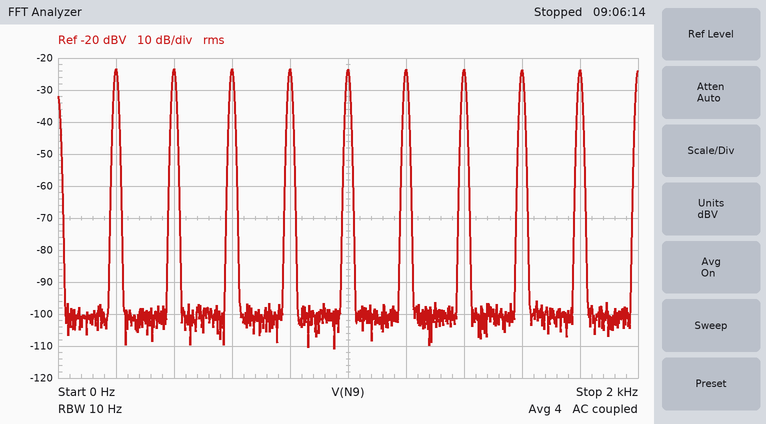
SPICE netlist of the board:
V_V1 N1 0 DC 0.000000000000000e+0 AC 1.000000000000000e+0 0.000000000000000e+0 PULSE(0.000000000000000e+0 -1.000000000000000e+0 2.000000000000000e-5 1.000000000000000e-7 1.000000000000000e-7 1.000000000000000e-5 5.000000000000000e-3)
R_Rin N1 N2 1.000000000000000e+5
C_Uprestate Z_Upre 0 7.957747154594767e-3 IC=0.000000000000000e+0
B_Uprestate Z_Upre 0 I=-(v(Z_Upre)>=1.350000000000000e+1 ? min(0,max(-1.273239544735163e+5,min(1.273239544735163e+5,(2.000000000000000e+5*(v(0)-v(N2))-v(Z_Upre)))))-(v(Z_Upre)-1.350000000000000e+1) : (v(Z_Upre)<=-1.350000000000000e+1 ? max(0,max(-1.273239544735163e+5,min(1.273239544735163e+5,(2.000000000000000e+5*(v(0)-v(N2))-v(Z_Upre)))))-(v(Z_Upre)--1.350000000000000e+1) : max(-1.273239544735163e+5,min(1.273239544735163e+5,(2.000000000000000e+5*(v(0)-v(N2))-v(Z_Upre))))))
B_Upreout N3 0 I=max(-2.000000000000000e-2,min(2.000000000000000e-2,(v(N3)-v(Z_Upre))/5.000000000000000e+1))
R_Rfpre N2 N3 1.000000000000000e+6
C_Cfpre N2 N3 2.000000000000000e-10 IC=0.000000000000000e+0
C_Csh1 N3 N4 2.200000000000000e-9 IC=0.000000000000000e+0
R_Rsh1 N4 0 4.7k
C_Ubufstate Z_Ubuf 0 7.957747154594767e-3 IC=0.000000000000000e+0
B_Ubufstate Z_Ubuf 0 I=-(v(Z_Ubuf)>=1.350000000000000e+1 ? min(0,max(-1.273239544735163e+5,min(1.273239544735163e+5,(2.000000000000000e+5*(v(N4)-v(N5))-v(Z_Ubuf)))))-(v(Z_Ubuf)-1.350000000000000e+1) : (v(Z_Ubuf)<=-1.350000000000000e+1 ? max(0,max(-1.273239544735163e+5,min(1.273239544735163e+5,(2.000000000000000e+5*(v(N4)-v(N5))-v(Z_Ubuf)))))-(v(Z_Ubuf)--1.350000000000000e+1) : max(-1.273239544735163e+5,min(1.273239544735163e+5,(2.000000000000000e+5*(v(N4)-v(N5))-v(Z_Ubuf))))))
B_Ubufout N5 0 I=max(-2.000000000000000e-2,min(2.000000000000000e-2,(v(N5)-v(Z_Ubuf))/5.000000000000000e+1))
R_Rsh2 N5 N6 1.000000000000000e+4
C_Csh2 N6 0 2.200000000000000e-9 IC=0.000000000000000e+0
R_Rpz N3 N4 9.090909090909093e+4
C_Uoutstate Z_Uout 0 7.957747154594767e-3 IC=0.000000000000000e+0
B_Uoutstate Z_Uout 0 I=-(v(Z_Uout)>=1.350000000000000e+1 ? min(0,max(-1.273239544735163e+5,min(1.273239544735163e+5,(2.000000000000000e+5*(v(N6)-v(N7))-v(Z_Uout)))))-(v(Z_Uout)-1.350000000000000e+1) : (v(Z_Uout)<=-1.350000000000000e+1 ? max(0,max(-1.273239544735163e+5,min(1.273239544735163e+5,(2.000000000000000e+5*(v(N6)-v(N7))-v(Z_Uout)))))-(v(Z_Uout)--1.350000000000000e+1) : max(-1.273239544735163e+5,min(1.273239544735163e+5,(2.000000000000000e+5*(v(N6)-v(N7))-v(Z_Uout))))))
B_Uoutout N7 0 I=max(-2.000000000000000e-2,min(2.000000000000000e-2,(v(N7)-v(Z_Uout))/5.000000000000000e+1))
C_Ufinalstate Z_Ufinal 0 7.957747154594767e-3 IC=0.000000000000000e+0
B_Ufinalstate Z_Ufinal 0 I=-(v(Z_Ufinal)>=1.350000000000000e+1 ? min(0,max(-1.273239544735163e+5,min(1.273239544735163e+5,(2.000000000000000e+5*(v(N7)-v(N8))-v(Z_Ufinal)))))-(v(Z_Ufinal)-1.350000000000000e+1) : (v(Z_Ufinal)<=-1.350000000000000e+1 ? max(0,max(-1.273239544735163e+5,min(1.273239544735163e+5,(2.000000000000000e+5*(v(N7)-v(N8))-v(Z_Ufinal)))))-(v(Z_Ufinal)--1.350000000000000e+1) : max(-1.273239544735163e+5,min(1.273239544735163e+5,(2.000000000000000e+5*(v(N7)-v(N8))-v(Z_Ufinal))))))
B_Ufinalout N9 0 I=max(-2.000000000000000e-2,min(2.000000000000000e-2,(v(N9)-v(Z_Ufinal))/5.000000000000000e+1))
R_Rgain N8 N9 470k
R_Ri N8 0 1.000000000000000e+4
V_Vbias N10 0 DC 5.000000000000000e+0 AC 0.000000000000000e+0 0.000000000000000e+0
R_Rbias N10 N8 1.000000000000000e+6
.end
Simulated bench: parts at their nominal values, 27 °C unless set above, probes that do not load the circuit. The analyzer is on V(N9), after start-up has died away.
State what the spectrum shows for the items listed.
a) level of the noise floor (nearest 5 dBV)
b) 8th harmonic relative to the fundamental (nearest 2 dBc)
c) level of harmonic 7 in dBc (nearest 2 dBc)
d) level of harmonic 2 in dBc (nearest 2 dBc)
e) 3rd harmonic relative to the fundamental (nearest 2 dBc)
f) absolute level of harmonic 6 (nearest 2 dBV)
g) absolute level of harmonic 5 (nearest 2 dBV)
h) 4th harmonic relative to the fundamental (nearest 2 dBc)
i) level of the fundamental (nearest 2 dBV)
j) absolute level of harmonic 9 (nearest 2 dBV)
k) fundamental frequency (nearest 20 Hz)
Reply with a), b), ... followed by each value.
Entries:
a) -100 dBV
b) 0 dBc
c) 0 dBc
d) 0 dBc
e) 0 dBc
f) -24 dBV
g) -24 dBV
h) 0 dBc
i) -24 dBV
j) -24 dBV
k) 200 Hz
